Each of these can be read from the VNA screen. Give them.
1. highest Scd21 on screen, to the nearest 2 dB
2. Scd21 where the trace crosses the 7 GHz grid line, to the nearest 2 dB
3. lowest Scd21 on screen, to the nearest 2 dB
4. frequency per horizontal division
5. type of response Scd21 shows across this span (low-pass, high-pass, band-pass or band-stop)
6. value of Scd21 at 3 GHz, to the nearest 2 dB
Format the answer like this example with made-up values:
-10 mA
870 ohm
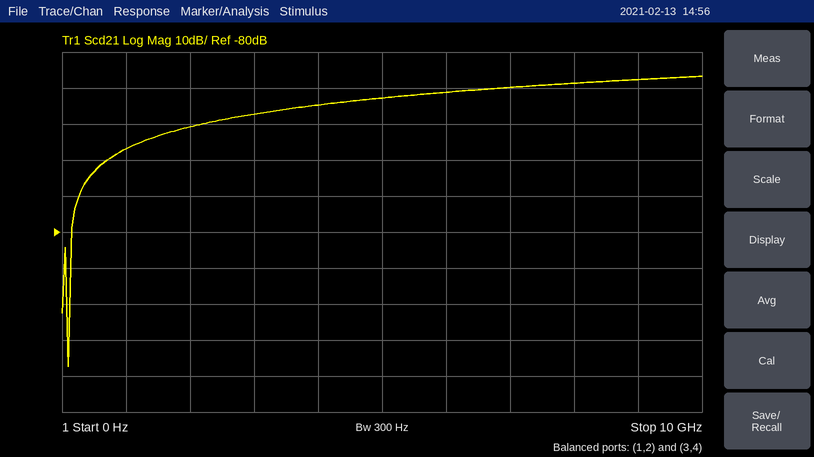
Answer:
-36 dB
-40 dB
-118 dB
1 GHz
high-pass
-48 dB
